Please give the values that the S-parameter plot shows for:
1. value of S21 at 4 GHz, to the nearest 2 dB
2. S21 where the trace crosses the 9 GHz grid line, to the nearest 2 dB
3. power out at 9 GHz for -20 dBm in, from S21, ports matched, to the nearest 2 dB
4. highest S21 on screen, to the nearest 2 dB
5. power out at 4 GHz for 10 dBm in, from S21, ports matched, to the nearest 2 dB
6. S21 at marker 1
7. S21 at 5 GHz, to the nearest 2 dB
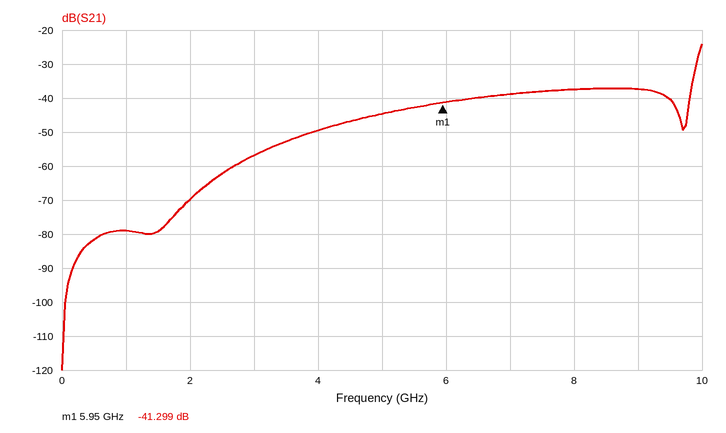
-50 dB
-38 dB
-58 dBm
-24 dB
-40 dBm
-41.299 dB
-44 dB
